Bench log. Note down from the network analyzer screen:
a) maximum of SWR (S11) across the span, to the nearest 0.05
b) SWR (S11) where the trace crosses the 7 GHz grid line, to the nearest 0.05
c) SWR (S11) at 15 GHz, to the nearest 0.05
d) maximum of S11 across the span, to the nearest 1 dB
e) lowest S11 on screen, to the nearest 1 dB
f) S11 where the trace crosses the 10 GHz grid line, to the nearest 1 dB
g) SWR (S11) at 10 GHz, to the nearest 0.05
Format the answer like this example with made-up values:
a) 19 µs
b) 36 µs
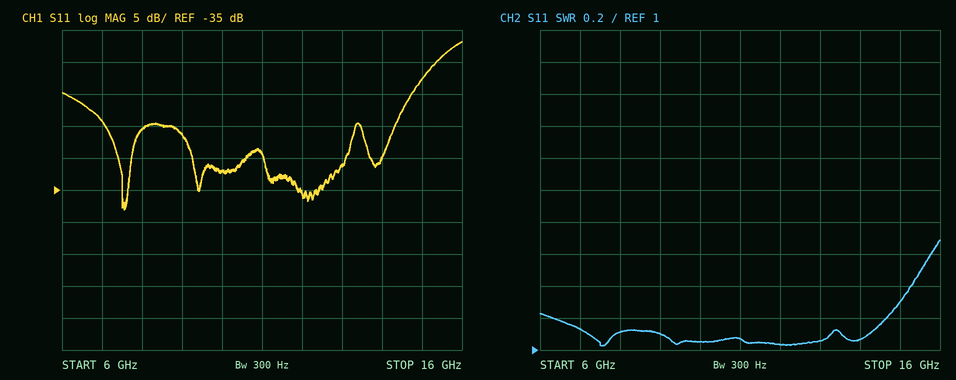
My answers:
a) 1.70
b) 1.15
c) 1.30
d) -12 dB
e) -38 dB
f) -32 dB
g) 1.05
